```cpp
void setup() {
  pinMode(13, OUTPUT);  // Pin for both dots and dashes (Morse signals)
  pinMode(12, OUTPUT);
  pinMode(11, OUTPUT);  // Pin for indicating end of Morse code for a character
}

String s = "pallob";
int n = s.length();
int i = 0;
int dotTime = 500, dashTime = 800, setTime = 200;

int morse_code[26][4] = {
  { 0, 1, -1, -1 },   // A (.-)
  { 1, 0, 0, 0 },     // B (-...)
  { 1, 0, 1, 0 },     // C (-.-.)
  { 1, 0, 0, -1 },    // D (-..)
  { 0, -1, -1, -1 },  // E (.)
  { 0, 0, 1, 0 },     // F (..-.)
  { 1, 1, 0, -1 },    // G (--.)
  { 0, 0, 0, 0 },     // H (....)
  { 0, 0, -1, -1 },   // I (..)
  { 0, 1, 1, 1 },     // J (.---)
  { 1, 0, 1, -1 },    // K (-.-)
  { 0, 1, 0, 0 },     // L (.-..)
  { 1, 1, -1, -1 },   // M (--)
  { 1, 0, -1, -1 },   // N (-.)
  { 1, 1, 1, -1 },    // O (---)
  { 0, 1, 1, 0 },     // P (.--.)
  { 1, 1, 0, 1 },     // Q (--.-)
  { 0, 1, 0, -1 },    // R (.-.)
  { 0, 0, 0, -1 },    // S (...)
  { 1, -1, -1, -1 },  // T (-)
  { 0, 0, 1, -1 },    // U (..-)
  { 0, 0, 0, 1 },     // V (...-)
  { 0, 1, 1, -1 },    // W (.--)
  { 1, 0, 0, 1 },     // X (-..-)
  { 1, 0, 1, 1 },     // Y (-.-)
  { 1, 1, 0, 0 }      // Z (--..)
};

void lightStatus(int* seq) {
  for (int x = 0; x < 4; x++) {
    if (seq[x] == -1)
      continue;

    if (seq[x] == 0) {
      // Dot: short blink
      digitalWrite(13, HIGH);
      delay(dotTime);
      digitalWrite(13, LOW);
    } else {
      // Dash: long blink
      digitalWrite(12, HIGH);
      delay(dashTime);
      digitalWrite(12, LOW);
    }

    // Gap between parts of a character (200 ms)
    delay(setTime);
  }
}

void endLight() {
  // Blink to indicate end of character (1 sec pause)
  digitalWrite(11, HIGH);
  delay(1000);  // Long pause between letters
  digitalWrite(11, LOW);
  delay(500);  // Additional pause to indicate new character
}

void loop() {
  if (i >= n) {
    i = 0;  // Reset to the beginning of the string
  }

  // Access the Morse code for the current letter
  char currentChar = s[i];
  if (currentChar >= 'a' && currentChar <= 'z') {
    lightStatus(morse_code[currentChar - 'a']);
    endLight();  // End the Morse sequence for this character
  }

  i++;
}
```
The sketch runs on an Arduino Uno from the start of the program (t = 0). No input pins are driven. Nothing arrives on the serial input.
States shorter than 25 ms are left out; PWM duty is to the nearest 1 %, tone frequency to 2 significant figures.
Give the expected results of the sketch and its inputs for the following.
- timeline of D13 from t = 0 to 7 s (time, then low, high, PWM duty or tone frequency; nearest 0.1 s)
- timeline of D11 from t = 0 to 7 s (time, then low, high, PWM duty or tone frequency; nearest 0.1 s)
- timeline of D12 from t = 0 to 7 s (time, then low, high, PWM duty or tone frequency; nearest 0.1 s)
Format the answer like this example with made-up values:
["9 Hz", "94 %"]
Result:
["0 s high; 0.5 s low; 2.7 s high; 3.2 s low; 4.9 s high; 5.4 s low", "0 s low; 3.4 s high; 4.4 s low; 6.6 s high", "0 s low; 0.7 s high; 1.5 s low; 1.7 s high; 2.5 s low; 5.6 s high; 6.4 s low"]
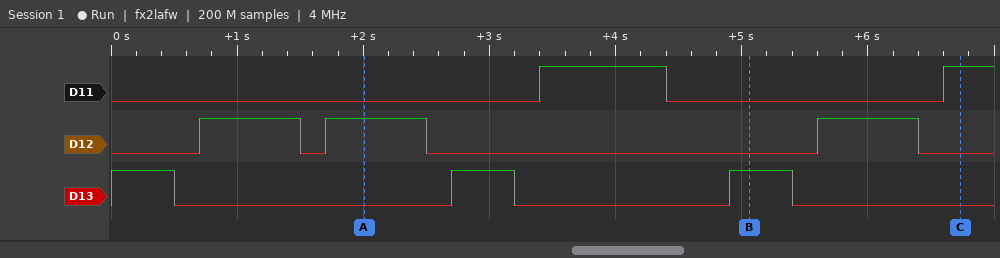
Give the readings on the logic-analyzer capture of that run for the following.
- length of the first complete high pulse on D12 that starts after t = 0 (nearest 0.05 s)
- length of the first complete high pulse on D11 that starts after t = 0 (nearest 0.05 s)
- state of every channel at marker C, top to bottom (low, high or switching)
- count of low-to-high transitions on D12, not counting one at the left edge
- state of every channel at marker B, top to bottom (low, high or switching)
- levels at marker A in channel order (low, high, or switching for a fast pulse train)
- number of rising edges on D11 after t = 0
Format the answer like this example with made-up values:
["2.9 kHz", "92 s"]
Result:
["0.80 s", "1.00 s", "D11 high, D12 low, D13 low", "3", "D11 low, D12 low, D13 high", "D11 low, D12 high, D13 low", "2"]
